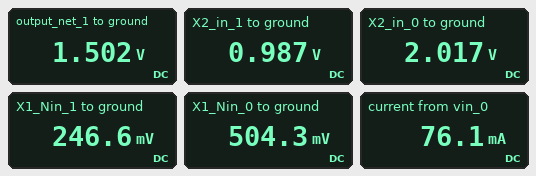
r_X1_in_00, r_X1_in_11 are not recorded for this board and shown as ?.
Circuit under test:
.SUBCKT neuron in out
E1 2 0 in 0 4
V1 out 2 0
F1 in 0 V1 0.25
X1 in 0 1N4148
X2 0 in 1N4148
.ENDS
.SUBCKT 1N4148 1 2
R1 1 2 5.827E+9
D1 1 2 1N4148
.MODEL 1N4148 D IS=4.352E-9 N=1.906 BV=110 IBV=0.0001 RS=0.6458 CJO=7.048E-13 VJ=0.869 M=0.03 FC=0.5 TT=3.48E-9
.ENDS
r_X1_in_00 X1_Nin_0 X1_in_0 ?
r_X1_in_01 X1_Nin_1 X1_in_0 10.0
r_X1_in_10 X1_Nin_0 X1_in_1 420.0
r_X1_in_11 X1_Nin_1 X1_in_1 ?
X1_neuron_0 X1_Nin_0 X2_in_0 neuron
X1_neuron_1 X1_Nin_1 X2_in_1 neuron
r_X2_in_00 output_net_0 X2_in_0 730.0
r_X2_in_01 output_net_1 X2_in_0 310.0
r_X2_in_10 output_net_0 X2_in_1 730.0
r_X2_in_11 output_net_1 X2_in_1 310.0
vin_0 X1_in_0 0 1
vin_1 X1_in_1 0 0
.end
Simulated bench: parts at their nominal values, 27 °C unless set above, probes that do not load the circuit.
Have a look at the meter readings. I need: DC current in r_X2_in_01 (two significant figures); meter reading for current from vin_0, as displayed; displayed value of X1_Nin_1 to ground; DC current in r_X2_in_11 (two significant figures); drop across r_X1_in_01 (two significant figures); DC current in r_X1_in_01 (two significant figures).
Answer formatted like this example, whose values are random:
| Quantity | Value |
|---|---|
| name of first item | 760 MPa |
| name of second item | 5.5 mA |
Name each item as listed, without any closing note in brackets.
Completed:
| Quantity | Value |
|---|---|
| DC current in r_X2_in_01 | 1.7 mA |
| meter reading for current from vin_0, as displayed | 76.1 mA |
| displayed value of X1_Nin_1 to ground | 246.6 mV |
| DC current in r_X2_in_11 | 1.7 mA |
| drop across r_X1_in_01 | 750 mV |
| DC current in r_X1_in_01 | 75 mA |
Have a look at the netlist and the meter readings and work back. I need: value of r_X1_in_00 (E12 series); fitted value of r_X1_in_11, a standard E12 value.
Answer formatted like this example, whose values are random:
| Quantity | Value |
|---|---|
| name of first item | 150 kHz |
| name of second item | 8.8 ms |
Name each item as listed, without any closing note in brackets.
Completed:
| Quantity | Value |
|---|---|
| value of r_X1_in_00 | 680 Ω |
| fitted value of r_X1_in_11, a standard E12 value | 3.3 Ω |
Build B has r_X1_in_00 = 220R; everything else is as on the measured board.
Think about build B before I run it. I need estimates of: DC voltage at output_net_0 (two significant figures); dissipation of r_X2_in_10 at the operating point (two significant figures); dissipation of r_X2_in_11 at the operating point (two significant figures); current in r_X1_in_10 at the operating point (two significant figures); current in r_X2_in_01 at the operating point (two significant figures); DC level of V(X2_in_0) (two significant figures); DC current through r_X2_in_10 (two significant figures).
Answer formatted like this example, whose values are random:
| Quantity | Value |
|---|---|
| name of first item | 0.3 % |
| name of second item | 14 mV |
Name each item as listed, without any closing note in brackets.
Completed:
| Quantity | Value |
|---|---|
| DC voltage at output_net_0 | 1.7 V |
| dissipation of r_X2_in_10 at the operating point | 750 µW |
| dissipation of r_X2_in_11 at the operating point | 1.8 mW |
| current in r_X1_in_10 at the operating point | 1.5 mA |
| current in r_X2_in_01 at the operating point | 2.4 mA |
| DC level of V(X2_in_0) | 2.5 V |
| DC current through r_X2_in_10 | 1.0 mA |
